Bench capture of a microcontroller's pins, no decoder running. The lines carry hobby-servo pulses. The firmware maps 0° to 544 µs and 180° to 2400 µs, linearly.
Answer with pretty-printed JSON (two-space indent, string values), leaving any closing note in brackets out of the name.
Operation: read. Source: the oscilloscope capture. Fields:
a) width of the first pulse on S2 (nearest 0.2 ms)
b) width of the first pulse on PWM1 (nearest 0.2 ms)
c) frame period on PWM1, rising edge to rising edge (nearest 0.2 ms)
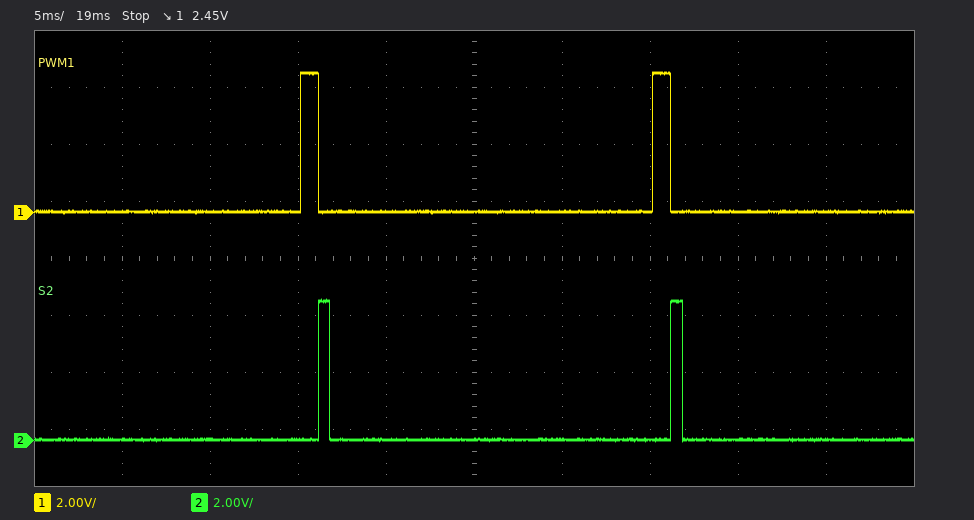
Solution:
{
  "width of the first pulse on S2": "0.6 ms",
  "width of the first pulse on PWM1": "1.0 ms",
  "frame period on PWM1, rising edge to rising edge": "20.0 ms"
}
